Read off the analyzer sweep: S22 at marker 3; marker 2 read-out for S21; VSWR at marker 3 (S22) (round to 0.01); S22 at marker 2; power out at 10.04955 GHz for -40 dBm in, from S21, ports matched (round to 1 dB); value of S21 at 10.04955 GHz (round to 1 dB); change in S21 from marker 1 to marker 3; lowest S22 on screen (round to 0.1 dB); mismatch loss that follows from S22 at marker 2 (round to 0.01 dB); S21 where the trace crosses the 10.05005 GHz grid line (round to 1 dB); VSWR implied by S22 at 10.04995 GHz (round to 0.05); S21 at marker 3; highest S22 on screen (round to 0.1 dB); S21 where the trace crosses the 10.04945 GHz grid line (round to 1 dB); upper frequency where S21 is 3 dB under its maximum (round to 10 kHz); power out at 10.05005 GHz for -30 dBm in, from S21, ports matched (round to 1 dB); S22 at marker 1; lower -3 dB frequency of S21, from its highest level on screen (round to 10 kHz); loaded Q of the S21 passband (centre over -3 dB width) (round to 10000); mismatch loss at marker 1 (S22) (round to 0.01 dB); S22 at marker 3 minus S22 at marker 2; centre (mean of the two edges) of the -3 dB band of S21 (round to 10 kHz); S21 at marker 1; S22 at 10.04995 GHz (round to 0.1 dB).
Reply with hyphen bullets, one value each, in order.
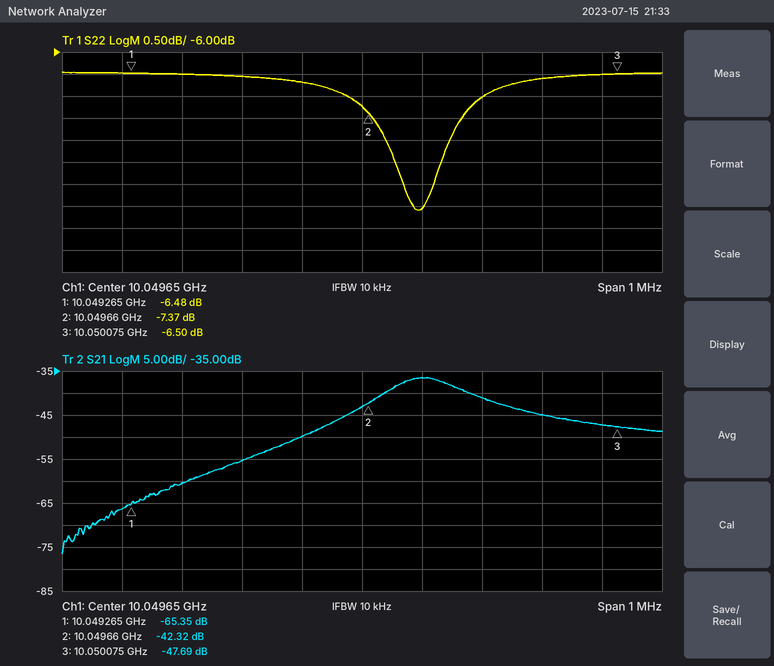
- -6.50 dB
- -42.32 dB
- 2.80
- -7.37 dB
- -90 dBm
- -50 dB
- 17.66 dB
- -9.6 dB
- 0.88 dB
- -47 dB
- 2.75
- -47.69 dB
- -6.5 dB
- -55 dB
- 10.04982 GHz
- -77 dBm
- -6.48 dB
- 10.04969 GHz
- 80000
- 1.11 dB
- 0.87 dB
- 10.04976 GHz
- -65.35 dB
- -6.6 dB
